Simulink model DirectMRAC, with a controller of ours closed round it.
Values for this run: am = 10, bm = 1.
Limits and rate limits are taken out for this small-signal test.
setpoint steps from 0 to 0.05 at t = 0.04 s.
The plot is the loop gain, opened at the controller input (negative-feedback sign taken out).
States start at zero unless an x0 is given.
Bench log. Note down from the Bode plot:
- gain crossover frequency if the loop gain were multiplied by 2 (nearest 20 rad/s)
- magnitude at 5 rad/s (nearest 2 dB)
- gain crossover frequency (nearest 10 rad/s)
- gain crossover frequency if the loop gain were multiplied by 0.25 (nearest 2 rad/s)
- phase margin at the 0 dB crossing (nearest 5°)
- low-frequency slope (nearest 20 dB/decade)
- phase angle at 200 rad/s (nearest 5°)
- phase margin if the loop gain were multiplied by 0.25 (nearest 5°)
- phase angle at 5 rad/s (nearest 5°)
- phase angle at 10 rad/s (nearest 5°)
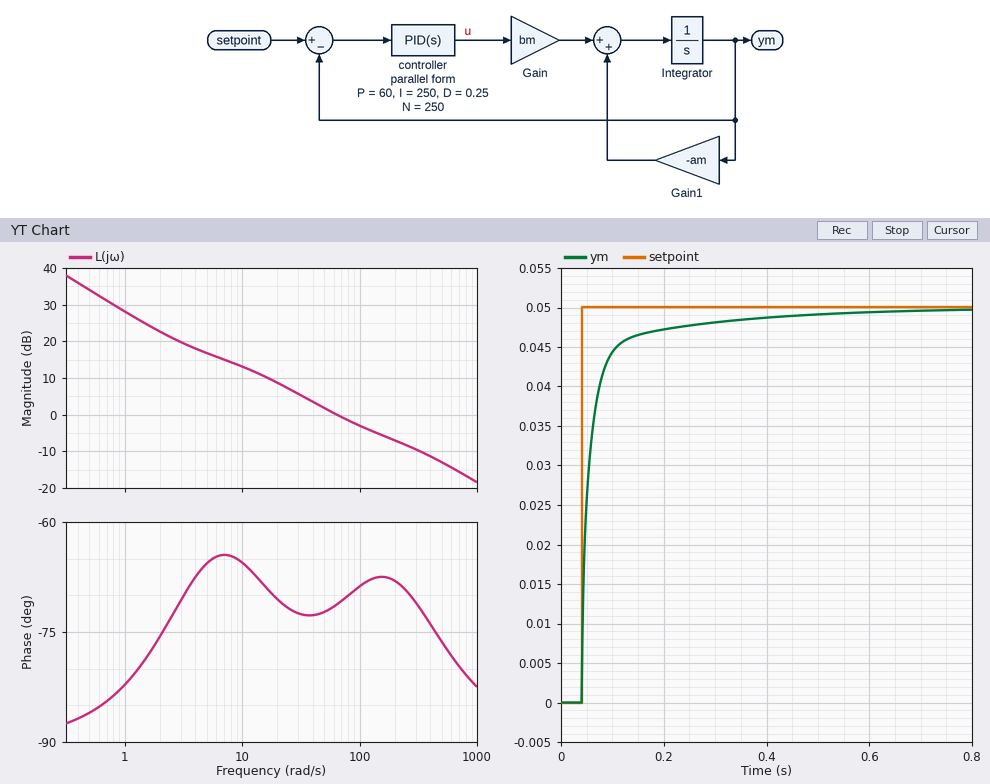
160 rad/s
16 dB
60 rad/s
12 rad/s
110°
-20 dB/decade
-70°
115°
-65°
-65°
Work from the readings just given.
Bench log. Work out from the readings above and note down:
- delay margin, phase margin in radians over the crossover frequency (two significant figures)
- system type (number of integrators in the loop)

0.032 s
1
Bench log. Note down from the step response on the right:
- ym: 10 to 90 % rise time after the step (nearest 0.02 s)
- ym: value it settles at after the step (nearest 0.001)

0.06 s
0.050
